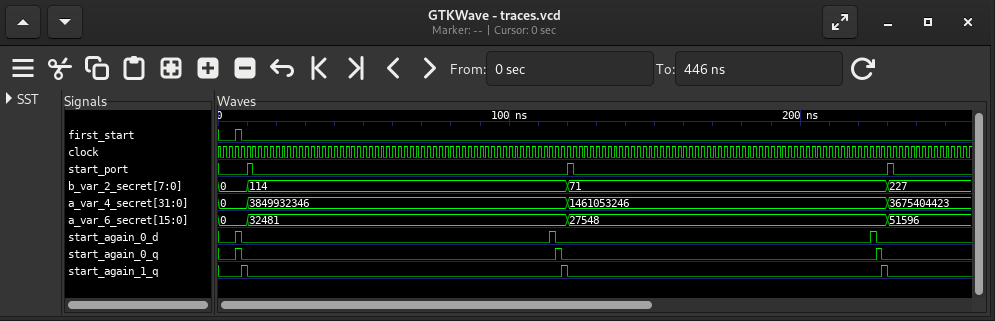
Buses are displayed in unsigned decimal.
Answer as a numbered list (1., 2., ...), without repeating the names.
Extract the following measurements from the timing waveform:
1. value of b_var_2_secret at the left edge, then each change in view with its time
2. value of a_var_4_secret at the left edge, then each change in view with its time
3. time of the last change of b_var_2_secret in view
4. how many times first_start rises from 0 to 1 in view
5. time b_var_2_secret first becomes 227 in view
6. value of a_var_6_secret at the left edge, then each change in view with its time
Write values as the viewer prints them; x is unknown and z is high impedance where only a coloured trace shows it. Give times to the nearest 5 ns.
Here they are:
1. 0, 114 at 10 ns, 71 at 120 ns, 227 at 230 ns
2. 0, 3849932346 at 10 ns, 1461053246 at 120 ns, 3675404423 at 230 ns
3. 230 ns
4. 1
5. 230 ns
6. 0, 32481 at 10 ns, 27548 at 120 ns, 51596 at 230 ns
